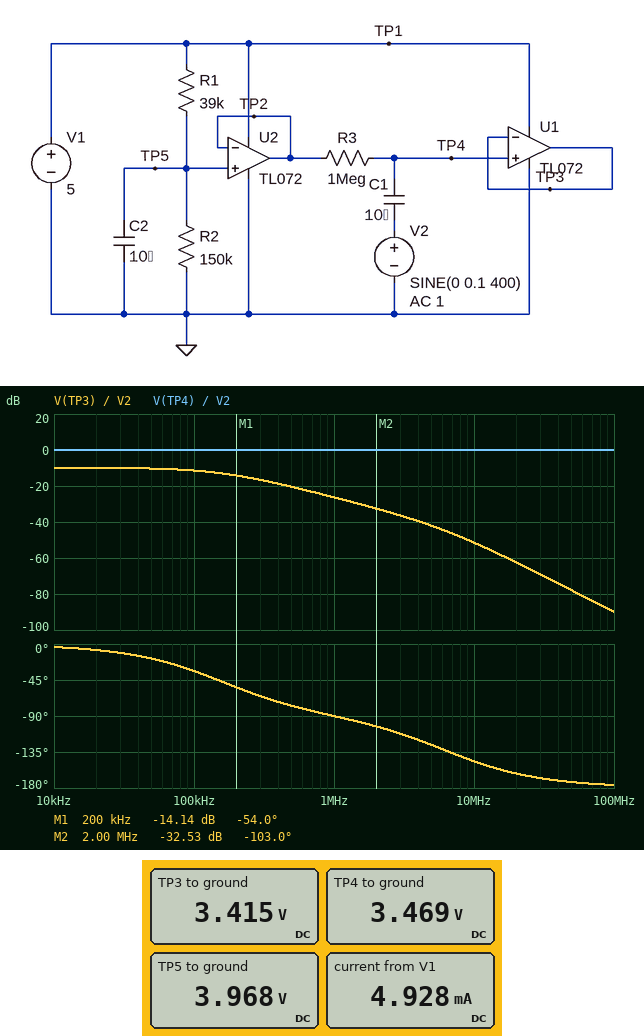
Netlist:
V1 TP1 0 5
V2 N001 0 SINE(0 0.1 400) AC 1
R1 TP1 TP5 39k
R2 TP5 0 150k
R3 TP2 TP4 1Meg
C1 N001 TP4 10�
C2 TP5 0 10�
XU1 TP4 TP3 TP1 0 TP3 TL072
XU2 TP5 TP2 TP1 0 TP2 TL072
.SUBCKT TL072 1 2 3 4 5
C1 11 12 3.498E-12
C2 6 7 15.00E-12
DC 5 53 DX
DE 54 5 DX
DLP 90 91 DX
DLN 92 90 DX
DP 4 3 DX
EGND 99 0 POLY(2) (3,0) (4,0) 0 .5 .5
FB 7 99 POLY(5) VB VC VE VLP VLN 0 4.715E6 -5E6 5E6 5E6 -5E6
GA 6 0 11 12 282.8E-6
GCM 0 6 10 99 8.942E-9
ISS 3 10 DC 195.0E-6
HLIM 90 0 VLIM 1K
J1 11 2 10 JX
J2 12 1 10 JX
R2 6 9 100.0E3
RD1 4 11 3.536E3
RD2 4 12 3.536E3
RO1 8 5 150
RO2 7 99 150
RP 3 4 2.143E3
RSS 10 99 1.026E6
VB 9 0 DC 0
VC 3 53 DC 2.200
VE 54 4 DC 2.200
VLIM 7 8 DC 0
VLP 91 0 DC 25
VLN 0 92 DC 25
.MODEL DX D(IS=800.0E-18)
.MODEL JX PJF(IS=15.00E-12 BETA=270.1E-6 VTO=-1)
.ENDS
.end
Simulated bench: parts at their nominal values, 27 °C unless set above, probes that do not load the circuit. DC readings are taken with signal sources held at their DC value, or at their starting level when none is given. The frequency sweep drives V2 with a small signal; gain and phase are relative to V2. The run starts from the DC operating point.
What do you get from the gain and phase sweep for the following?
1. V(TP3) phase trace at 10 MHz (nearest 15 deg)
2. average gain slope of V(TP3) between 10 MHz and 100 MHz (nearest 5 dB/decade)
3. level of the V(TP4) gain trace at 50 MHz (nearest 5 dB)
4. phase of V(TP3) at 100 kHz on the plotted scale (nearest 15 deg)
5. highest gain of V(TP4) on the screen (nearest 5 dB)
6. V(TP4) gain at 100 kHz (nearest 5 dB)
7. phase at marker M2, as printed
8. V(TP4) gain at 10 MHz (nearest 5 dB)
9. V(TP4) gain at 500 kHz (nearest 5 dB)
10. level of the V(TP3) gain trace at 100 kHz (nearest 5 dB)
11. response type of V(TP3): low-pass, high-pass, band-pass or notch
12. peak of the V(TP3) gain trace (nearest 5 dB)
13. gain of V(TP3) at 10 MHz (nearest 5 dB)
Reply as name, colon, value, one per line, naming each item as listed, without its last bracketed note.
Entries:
V(TP3) phase trace at 10 MHz: -150 deg
average gain slope of V(TP3) between 10 MHz and 100 MHz: -40 dB/decade
level of the V(TP4) gain trace at 50 MHz: 0 dB
phase of V(TP3) at 100 kHz on the plotted scale: -30 deg
highest gain of V(TP4) on the screen: 0 dB
V(TP4) gain at 100 kHz: 0 dB
phase at marker M2, as printed: -103.0 deg
V(TP4) gain at 10 MHz: 0 dB
V(TP4) gain at 500 kHz: 0 dB
level of the V(TP3) gain trace at 100 kHz: -10 dB
response type of V(TP3): low-pass, high-pass, band-pass or notch: low-pass
peak of the V(TP3) gain trace: -10 dB
gain of V(TP3) at 10 MHz: -50 dB
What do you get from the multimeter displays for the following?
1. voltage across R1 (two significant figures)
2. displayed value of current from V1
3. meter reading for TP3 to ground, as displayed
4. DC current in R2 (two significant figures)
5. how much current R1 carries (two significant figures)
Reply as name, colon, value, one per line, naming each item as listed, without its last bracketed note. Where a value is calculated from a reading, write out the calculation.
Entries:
voltage across R1: 5 V - 3.968 V = 1.0 V
displayed value of current from V1: 4.928 mA
meter reading for TP3 to ground, as displayed: 3.415 V
DC current in R2: (3.968 V) / 150 kΩ = 26 µA
how much current R1 carries: (5 V - 3.968 V) / 39 kΩ = 26 µA
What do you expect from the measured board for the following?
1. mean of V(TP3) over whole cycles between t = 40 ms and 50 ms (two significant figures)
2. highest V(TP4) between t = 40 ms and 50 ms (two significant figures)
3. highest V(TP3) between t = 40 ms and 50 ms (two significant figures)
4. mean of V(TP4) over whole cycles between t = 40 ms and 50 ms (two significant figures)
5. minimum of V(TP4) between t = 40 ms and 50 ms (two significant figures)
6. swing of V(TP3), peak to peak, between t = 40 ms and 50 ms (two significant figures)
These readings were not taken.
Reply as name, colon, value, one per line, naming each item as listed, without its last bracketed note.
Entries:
mean of V(TP3) over whole cycles between t = 40 ms and 50 ms: 3.4 V
highest V(TP4) between t = 40 ms and 50 ms: 3.6 V
highest V(TP3) between t = 40 ms and 50 ms: 3.4 V
mean of V(TP4) over whole cycles between t = 40 ms and 50 ms: 3.5 V
minimum of V(TP4) between t = 40 ms and 50 ms: 3.4 V
swing of V(TP3), peak to peak, between t = 40 ms and 50 ms: 75 mV
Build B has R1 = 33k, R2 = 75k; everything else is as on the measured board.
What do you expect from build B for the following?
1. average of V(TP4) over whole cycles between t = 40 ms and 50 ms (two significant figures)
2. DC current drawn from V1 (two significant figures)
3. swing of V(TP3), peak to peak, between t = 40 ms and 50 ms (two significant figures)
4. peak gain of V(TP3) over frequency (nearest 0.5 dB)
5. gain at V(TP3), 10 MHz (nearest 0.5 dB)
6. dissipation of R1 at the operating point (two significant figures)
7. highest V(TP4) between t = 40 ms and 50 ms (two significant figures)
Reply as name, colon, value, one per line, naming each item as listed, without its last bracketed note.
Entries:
average of V(TP4) over whole cycles between t = 40 ms and 50 ms: 3.4 V
DC current drawn from V1: 5.1 mA
swing of V(TP3), peak to peak, between t = 40 ms and 50 ms: 110 mV
peak gain of V(TP3) over frequency: -5.5 dB
gain at V(TP3), 10 MHz: -44.0 dB
dissipation of R1 at the operating point: 71 µW
highest V(TP4) between t = 40 ms and 50 ms: 3.5 V
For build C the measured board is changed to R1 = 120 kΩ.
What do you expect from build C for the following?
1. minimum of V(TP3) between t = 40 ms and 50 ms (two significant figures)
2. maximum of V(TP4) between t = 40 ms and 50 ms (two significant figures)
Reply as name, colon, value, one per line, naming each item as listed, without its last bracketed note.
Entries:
minimum of V(TP3) between t = 40 ms and 50 ms: 2.7 V
maximum of V(TP4) between t = 40 ms and 50 ms: 2.9 V
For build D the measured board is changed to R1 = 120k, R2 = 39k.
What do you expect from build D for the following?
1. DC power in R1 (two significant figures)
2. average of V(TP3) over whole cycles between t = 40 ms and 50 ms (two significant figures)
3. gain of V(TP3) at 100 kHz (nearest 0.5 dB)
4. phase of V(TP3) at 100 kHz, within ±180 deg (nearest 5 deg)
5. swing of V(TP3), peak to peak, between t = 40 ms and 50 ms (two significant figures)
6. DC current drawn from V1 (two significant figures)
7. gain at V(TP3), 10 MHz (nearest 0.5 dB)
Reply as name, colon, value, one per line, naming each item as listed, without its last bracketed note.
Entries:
DC power in R1: 120 µW
average of V(TP3) over whole cycles between t = 40 ms and 50 ms: 1.6 V
gain of V(TP3) at 100 kHz: -10.0 dB
phase of V(TP3) at 100 kHz, within ±180 deg: -30 deg
swing of V(TP3), peak to peak, between t = 40 ms and 50 ms: 84 mV
DC current drawn from V1: 5.1 mA
gain at V(TP3), 10 MHz: -50.0 dB
